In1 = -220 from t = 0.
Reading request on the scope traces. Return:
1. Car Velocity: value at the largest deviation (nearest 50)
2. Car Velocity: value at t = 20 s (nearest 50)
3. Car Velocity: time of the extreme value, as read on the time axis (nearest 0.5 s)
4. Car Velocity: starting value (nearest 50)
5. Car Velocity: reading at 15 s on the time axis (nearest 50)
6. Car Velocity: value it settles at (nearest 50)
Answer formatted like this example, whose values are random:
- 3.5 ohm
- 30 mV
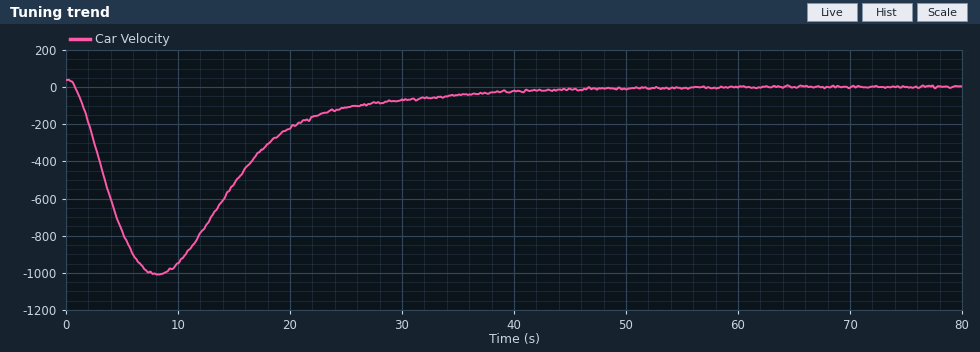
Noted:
- -1000
- -200
- 8.0 s
- 50
- -500
- 0
